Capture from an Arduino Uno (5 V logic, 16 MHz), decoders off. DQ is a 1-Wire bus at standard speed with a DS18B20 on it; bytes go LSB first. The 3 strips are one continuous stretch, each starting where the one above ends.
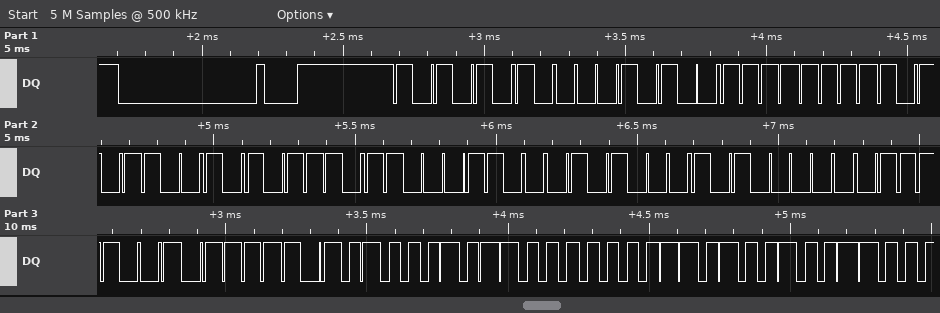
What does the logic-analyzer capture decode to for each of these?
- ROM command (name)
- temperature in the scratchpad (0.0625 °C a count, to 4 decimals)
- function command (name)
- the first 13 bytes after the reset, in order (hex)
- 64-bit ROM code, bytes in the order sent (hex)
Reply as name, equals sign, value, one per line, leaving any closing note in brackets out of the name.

ROM command = Match ROM
temperature in the scratchpad = 26.1250 °C
function command = Read Scratchpad
the first 13 bytes after the reset, in order = 55 28 FF 35 75 63 14 05 9E BE A2 01 4B
64-bit ROM code, bytes in the order sent = 28 FF 35 75 63 14 05 9E
